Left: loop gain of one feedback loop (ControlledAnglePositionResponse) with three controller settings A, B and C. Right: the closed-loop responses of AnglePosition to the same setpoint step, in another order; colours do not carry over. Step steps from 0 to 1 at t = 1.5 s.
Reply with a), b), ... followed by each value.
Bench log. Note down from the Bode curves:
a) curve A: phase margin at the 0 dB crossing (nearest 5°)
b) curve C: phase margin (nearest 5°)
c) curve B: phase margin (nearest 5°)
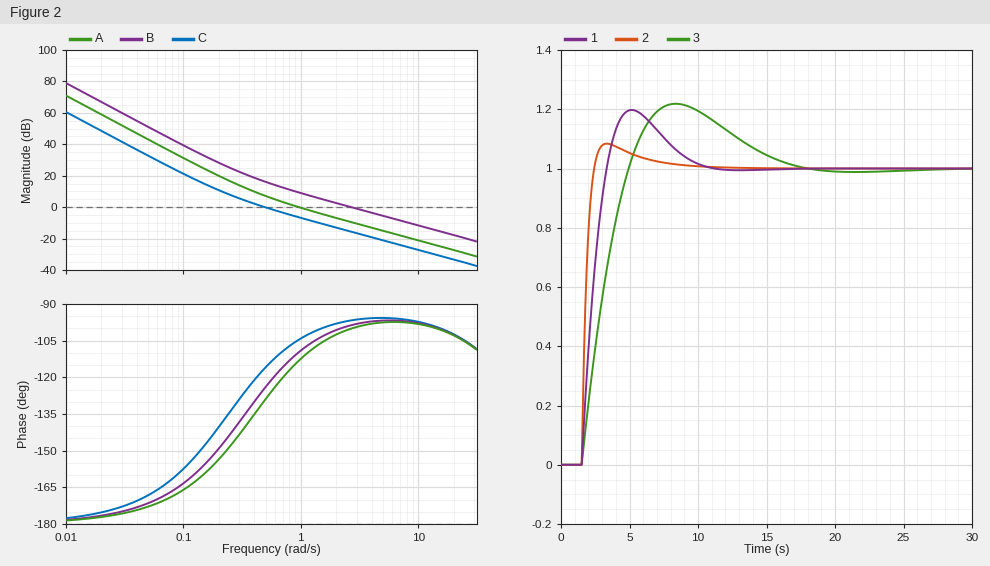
a) 65°
b) 65°
c) 80°
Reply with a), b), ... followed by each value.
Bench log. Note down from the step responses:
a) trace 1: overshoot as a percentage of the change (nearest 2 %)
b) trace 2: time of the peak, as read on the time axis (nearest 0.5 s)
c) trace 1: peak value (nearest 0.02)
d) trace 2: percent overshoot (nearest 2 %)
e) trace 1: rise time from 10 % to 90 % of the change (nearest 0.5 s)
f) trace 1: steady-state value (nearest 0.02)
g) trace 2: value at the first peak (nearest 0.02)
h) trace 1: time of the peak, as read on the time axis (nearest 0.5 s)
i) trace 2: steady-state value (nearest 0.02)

a) 20 %
b) 3.5 s
c) 1.20
d) 8 %
e) 1.5 s
f) 1.00
g) 1.08
h) 5.0 s
i) 1.00
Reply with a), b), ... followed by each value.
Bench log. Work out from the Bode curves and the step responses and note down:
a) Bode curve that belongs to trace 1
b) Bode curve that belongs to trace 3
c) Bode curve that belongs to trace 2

a) A
b) C
c) B
